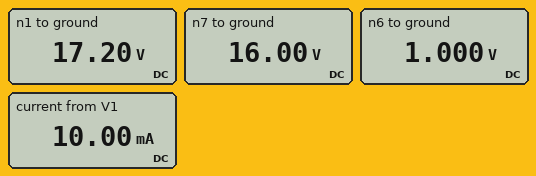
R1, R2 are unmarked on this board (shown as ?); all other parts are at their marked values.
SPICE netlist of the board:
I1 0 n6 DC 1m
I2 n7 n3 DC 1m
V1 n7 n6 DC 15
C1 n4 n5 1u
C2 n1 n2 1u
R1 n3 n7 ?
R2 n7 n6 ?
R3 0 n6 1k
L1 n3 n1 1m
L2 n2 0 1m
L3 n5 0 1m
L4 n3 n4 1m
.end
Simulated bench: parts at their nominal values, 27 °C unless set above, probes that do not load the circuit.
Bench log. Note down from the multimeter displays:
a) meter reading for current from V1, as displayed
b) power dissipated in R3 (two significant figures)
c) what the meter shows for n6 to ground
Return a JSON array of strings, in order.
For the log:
["10.00 mA", "1.0 mW", "1.000 V"]
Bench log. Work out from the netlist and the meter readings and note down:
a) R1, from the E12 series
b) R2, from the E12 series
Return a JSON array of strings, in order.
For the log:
["1.2 kΩ", "1.5 kΩ"]
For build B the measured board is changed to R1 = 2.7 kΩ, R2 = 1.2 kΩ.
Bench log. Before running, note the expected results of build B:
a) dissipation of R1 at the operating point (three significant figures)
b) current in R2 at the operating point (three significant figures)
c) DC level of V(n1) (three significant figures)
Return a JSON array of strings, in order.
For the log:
["2.70 mW", "12.5 mA", "18.7 V"]
